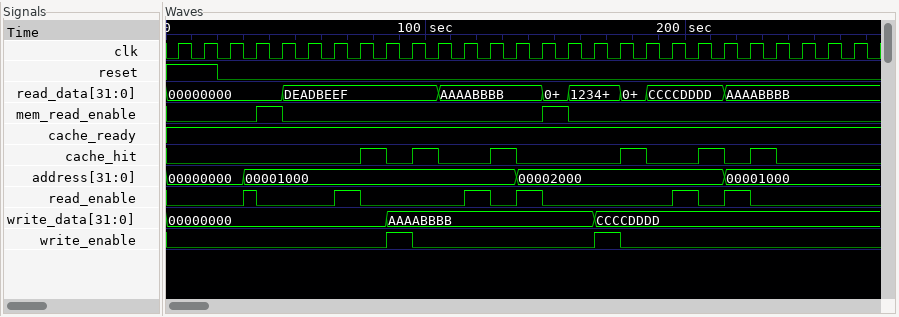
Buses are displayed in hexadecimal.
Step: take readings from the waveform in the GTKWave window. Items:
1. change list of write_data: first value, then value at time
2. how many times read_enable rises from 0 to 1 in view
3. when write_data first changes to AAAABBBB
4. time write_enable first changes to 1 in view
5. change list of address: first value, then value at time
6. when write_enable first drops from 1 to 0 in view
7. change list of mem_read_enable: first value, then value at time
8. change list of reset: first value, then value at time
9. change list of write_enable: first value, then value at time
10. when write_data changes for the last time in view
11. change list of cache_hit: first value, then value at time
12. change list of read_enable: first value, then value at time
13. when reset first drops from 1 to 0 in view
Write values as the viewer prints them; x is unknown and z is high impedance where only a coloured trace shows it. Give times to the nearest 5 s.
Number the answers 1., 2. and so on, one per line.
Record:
1. 00000000, AAAABBBB at 85 s, CCCCDDDD at 165 s
2. 6
3. 85 s
4. 85 s
5. 00000000, 00001000 at 30 s, 00002000 at 135 s, 00001000 at 215 s
6. 95 s
7. 0, 1 at 35 s, 0 at 45 s, 1 at 145 s, 0 at 155 s
8. 1, 0 at 20 s
9. 0, 1 at 85 s, 0 at 95 s, 1 at 165 s, 0 at 175 s
10. 165 s
11. 0, 1 at 75 s, 0 at 85 s, 1 at 95 s, 0 at 105 s, 1 at 125 s, 0 at 135 s, 1 at 175 s, 0 at 185 s, 1 at 205 s, 0 at 215 s, 1 at 225 s, 0 at 235 s
12. 0, 1 at 30 s, 0 at 35 s, 1 at 65 s, 0 at 75 s, 1 at 115 s, 0 at 125 s, 1 at 135 s, 0 at 145 s, 1 at 195 s, 0 at 205 s, 1 at 215 s, 0 at 225 s
13. 20 s
